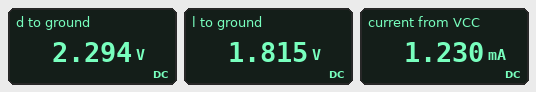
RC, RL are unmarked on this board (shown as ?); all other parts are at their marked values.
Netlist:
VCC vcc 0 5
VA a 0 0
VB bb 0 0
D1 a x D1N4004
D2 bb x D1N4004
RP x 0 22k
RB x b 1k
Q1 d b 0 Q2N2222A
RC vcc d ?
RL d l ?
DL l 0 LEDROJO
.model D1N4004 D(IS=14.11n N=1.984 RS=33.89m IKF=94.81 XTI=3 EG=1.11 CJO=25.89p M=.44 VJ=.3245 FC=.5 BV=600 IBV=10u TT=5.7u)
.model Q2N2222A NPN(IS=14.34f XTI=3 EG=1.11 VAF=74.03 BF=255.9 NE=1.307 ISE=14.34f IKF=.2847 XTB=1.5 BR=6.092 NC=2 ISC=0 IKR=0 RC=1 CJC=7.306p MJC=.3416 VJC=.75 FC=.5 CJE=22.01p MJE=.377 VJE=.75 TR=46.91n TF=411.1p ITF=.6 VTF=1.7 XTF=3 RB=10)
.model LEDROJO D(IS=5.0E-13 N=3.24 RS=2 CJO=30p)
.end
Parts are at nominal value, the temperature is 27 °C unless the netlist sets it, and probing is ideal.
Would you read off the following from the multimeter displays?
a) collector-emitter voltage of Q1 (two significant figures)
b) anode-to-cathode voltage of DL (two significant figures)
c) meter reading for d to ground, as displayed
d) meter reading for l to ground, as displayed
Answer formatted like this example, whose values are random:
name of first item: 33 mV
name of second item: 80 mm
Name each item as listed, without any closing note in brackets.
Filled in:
collector-emitter voltage of Q1: 2.3 V
anode-to-cathode voltage of DL: 1.8 V
meter reading for d to ground, as displayed: 2.294 V
meter reading for l to ground, as displayed: 1.815 V
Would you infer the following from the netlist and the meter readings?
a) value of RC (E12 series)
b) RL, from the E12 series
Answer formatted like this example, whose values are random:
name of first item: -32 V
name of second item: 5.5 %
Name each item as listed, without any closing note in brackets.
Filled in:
value of RC: 2.2 kΩ
RL, from the E12 series: 390 Ω
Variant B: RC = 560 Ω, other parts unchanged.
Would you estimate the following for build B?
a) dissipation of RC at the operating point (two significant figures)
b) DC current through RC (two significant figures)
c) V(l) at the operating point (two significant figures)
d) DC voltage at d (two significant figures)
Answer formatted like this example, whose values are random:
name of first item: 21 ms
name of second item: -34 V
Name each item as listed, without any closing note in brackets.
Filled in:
dissipation of RC at the operating point: 6.0 mW
DC current through RC: 3.3 mA
V(l) at the operating point: 1.9 V
DC voltage at d: 3.2 V
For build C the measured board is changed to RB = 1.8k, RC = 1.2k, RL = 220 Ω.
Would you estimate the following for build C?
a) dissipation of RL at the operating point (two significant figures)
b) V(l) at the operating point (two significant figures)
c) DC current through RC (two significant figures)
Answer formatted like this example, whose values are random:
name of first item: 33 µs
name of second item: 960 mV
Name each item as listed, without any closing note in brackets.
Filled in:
dissipation of RL at the operating point: 1.1 mW
V(l) at the operating point: 1.9 V
DC current through RC: 2.2 mA
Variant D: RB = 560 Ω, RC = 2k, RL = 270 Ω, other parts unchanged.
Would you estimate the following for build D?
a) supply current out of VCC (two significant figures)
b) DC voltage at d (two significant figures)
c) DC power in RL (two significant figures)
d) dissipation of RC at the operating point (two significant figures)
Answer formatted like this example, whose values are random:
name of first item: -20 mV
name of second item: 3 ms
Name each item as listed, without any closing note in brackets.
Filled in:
supply current out of VCC: 1.4 mA
DC voltage at d: 2.2 V
DC power in RL: 530 µW
dissipation of RC at the operating point: 3.9 mW
